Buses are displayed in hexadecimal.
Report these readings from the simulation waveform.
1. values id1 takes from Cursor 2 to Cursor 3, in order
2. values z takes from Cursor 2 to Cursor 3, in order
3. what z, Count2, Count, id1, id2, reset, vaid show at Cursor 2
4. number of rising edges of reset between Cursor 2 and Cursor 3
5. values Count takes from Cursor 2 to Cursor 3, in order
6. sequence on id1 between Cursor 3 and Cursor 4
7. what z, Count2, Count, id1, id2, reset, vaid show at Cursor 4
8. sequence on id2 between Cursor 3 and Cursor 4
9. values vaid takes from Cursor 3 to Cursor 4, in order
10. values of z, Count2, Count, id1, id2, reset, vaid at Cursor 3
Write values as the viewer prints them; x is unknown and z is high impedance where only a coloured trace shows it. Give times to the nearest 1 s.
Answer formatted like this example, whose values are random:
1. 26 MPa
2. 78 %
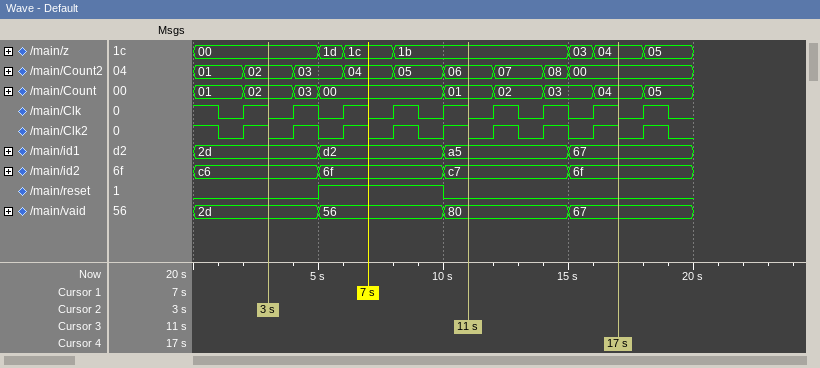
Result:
1. 2d, d2, a5
2. 00, 1d, 1c, 1b
3. z=00, Count2=02, Count=02, id1=2d, id2=c6, reset=0, vaid=2d
4. 1
5. 02, 03, 00, 01
6. a5, 67
7. z=04, Count2=00, Count=04, id1=67, id2=6f, reset=0, vaid=67
8. c7, 6f
9. 80, 67
10. z=1b, Count2=06, Count=01, id1=a5, id2=c7, reset=0, vaid=80
